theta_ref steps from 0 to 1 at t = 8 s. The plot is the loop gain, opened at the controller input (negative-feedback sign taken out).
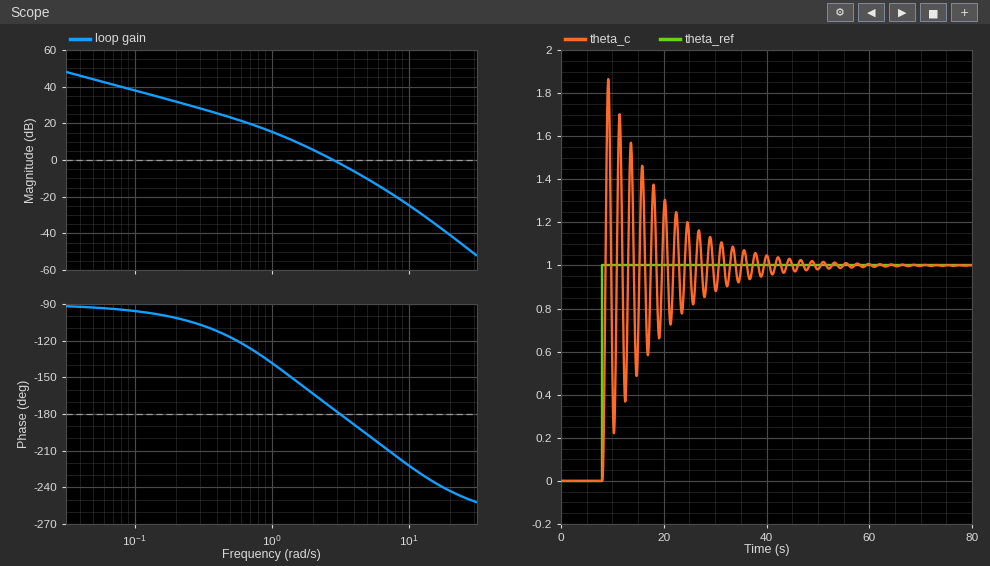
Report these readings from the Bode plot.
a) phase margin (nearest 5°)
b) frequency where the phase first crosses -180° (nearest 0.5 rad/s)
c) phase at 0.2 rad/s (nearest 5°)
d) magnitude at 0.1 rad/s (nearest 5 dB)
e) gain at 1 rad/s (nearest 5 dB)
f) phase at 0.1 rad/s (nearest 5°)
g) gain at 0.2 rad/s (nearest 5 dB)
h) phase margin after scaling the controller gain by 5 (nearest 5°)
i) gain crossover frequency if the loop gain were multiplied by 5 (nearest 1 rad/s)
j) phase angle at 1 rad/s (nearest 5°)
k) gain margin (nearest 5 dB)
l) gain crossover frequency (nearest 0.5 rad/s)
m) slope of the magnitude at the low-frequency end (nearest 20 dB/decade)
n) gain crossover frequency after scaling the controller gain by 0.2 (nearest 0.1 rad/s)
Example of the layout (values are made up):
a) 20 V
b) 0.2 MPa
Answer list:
a) 5°
b) 3.0 rad/s
c) -100°
d) 40 dB
e) 15 dB
f) -95°
g) 30 dB
h) -25°
i) 6 rad/s
j) -140°
k) 0 dB
l) 3.0 rad/s
m) -20 dB/decade
n) 1.1 rad/s
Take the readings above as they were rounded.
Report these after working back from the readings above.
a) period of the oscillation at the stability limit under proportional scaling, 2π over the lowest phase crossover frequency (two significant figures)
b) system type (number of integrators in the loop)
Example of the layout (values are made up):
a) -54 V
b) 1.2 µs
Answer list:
a) 2.1 s
b) 1
